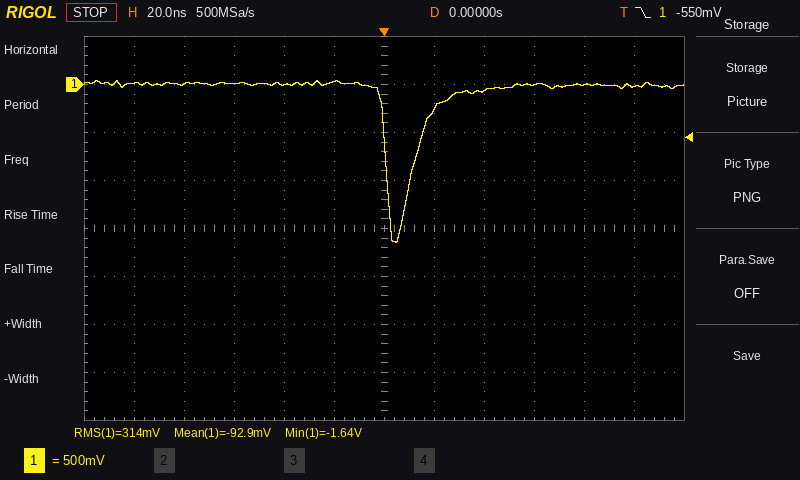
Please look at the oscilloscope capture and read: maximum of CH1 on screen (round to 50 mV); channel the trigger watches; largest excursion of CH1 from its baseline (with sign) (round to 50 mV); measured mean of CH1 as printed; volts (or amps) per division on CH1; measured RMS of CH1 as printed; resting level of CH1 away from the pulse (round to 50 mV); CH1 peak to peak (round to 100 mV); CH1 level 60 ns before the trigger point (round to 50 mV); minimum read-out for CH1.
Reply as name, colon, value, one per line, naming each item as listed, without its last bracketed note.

maximum of CH1 on screen: 50 mV
channel the trigger watches: CH1
largest excursion of CH1 from its baseline (with sign): -1.65 V
measured mean of CH1 as printed: -92.9 mV
volts (or amps) per division on CH1: 500 mV
measured RMS of CH1 as printed: 314 mV
resting level of CH1 away from the pulse: 0 mV
CH1 peak to peak: 1.70 V
CH1 level 60 ns before the trigger point: 0 mV
minimum read-out for CH1: -1.64 V
